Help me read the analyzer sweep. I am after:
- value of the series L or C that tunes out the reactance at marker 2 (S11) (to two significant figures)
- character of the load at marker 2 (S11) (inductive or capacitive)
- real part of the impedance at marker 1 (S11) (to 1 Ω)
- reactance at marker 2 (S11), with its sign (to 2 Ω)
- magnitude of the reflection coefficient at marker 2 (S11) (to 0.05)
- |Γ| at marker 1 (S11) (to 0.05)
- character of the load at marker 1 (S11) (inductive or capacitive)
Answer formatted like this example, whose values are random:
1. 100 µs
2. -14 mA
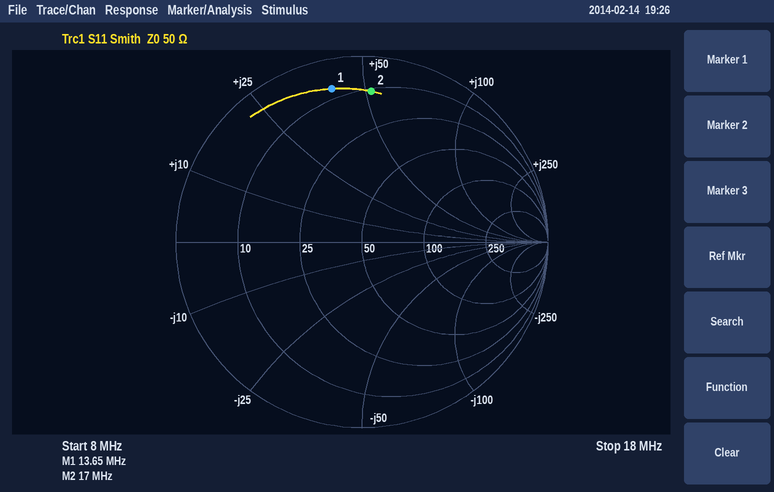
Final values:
1. 180 pF
2. inductive
3. 7 Ω
4. +52 Ω
5. 0.80
6. 0.85
7. inductive
